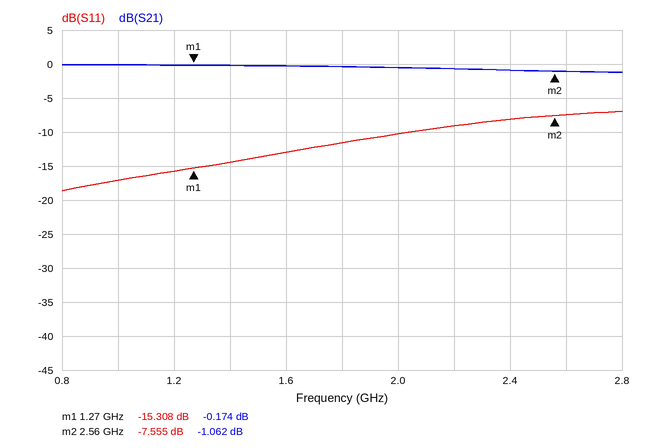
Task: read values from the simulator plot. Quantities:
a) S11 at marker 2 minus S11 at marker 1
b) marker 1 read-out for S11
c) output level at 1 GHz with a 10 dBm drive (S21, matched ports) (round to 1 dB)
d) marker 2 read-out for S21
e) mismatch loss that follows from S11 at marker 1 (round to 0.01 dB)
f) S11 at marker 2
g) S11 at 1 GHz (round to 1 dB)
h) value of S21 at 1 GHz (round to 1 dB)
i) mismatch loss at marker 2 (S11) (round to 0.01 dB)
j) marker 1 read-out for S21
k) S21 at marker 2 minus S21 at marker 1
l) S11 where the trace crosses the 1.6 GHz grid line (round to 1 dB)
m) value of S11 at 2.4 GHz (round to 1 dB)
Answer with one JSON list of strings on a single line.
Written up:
["7.753 dB", "-15.308 dB", "10 dBm", "-1.062 dB", "0.13 dB", "-7.555 dB", "-17 dB", "0 dB", "0.84 dB", "-0.174 dB", "-0.888 dB", "-13 dB", "-8 dB"]
